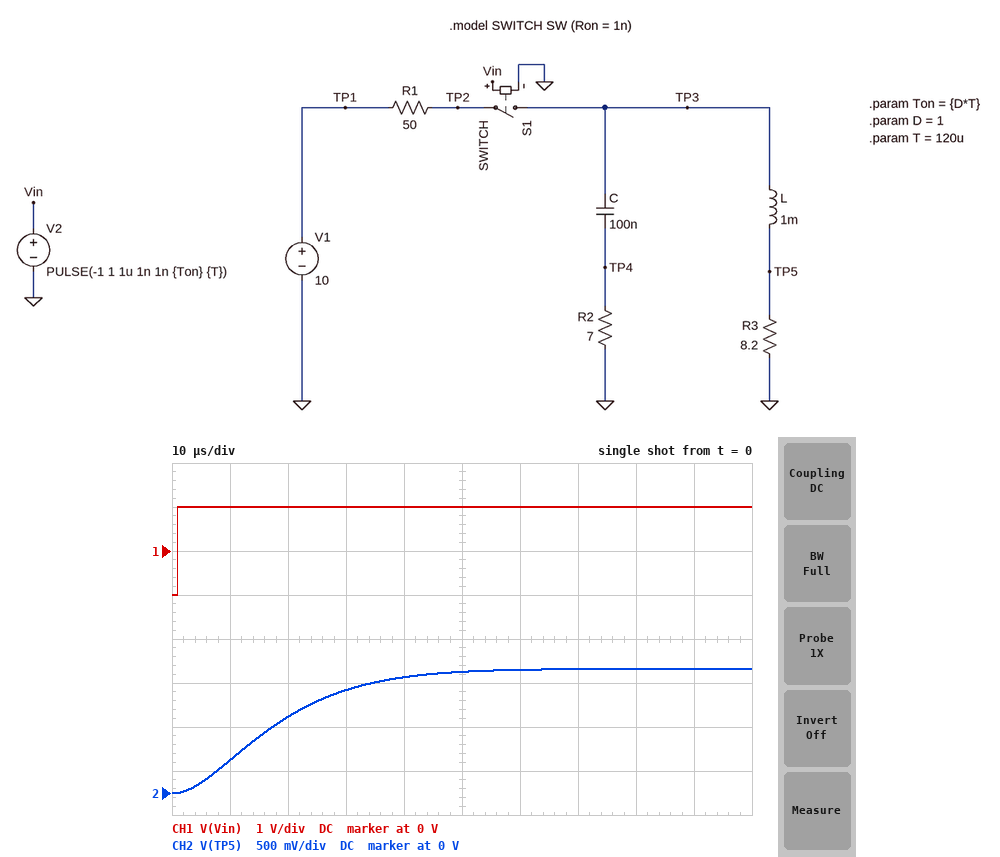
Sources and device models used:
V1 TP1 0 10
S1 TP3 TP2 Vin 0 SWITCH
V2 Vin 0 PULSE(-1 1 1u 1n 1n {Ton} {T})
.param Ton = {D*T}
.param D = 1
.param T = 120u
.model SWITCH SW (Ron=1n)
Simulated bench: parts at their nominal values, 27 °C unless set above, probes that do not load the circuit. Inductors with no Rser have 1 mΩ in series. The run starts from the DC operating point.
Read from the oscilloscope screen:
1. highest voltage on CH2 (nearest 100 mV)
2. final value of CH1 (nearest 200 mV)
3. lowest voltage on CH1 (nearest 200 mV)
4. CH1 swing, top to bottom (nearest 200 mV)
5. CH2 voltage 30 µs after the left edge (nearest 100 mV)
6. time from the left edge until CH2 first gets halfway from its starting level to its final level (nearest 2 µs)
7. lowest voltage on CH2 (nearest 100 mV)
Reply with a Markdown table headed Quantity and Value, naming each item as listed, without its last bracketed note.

| Quantity | Value |
|---|---|
| highest voltage on CH2 | 1.4 V |
| final value of CH1 | 1.0 V |
| lowest voltage on CH1 | -1.0 V |
| CH1 swing, top to bottom | 2.0 V |
| CH2 voltage 30 µs after the left edge | 1.2 V |
| time from the left edge until CH2 first gets halfway from its starting level to its final level | 16 µs |
| lowest voltage on CH2 | 0 V |
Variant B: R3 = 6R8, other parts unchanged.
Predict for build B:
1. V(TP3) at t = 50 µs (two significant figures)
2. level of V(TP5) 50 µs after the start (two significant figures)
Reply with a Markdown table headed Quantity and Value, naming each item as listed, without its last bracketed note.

| Quantity | Value |
|---|---|
| V(TP3) at t = 50 µs | 1.7 V |
| level of V(TP5) 50 µs after the start | 1.2 V |
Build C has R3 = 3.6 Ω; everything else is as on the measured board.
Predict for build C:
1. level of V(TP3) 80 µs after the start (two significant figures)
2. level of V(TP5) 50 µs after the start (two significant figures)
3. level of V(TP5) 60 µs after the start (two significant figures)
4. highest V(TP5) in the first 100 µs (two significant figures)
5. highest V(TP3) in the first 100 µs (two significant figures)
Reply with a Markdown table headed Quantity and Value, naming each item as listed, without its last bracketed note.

| Quantity | Value |
|---|---|
| level of V(TP3) 80 µs after the start | 700 mV |
| level of V(TP5) 50 µs after the start | 650 mV |
| level of V(TP5) 60 µs after the start | 660 mV |
| highest V(TP5) in the first 100 µs | 670 mV |
| highest V(TP3) in the first 100 µs | 7.1 V |
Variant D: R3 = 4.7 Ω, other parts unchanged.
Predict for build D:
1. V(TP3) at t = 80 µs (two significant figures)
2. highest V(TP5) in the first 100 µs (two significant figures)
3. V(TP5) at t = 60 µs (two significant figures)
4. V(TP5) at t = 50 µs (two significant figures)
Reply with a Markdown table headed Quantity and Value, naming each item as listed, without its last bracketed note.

| Quantity | Value |
|---|---|
| V(TP3) at t = 80 µs | 880 mV |
| highest V(TP5) in the first 100 µs | 860 mV |
| V(TP5) at t = 60 µs | 850 mV |
| V(TP5) at t = 50 µs | 830 mV |
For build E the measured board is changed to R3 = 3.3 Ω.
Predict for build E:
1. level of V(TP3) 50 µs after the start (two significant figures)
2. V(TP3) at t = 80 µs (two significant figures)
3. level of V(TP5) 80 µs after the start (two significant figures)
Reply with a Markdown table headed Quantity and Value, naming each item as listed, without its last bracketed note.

| Quantity | Value |
|---|---|
| level of V(TP3) 50 µs after the start | 1.2 V |
| V(TP3) at t = 80 µs | 650 mV |
| level of V(TP5) 80 µs after the start | 620 mV |
